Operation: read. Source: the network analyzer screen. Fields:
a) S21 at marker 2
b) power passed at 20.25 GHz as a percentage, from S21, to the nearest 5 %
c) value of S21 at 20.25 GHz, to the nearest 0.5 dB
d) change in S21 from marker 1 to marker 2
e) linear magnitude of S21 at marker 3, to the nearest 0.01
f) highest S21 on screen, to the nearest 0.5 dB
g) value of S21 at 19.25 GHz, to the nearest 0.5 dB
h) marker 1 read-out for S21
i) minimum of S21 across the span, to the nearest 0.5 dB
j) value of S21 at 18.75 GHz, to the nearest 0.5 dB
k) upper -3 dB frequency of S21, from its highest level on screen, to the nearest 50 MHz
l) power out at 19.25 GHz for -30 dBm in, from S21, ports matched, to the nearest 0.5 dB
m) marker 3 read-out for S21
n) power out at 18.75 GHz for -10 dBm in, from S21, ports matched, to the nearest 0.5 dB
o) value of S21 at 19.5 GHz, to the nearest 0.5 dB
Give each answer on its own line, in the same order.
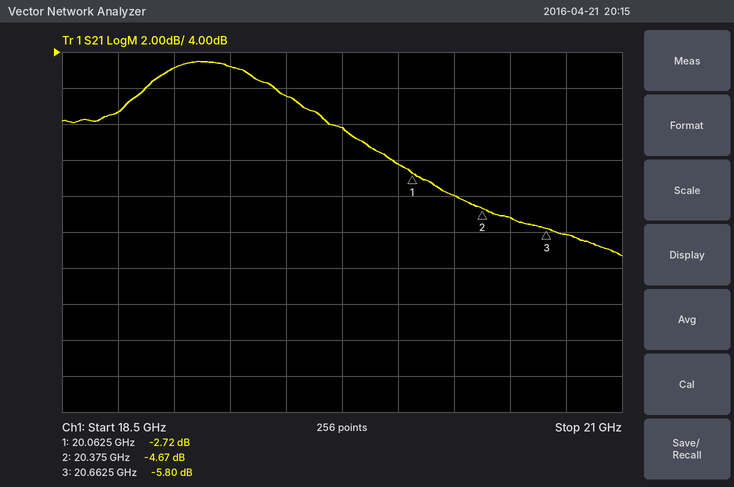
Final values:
-4.67 dB
40 %
-4.0 dB
-1.95 dB
0.51
3.5 dB
3.0 dB
-2.72 dB
-7.5 dB
0.5 dB
19.65 GHz
-27.0 dBm
-5.80 dB
-9.5 dBm
1.5 dB
